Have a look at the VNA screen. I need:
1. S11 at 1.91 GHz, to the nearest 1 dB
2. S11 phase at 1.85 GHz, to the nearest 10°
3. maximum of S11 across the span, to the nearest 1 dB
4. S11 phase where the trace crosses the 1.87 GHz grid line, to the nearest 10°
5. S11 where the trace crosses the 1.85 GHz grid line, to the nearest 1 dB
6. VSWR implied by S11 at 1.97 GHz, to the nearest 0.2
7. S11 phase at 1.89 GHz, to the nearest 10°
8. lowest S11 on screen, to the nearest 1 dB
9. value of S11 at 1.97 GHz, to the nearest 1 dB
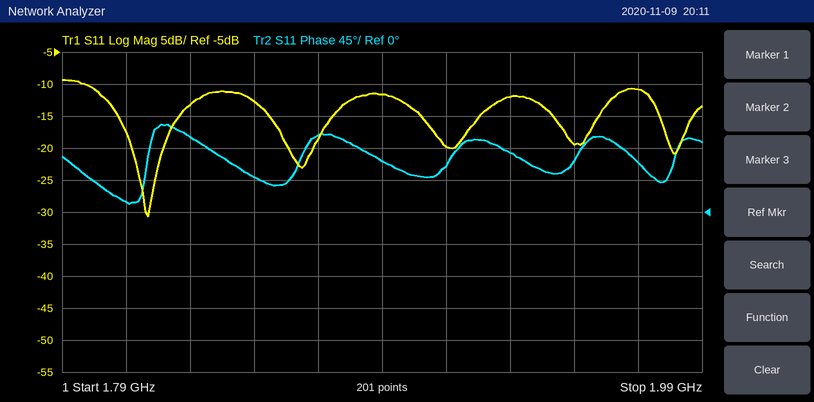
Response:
-20 dB
50°
-9 dB
110°
-13 dB
1.8
70°
-31 dB
-11 dB
